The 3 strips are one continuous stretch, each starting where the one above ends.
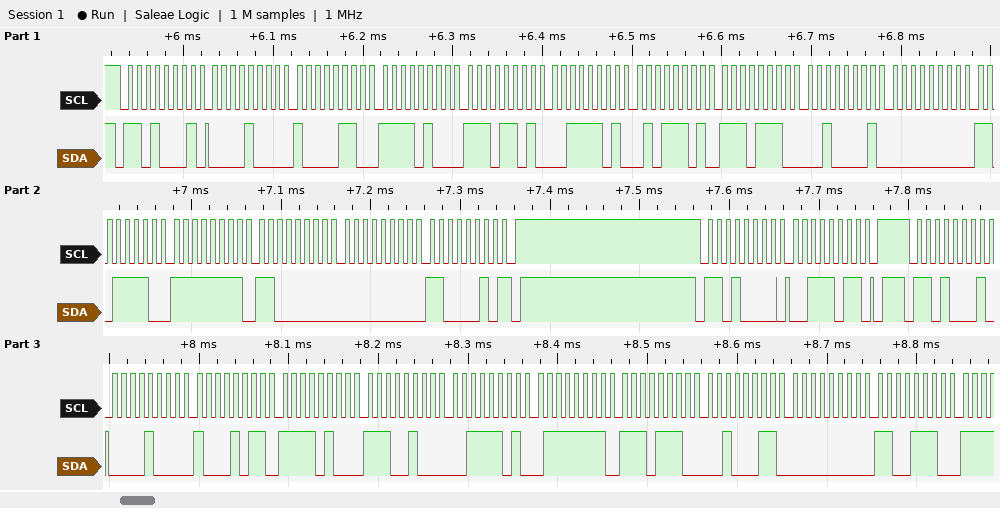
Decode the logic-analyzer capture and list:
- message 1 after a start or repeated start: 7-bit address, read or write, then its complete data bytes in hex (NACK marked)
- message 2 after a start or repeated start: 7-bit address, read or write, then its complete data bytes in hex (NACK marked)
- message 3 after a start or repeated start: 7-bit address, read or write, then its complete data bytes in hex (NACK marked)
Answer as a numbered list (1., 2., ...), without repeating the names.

1. 0x68 read: 08 86 F4 ED 3D 5D EE 21 00 DE FF C0 00 C2 NACK
2. 0x68 write: 3B
3. 0x68 read: 08 8B F4 E4 3D 7F EE 23 00 CE
